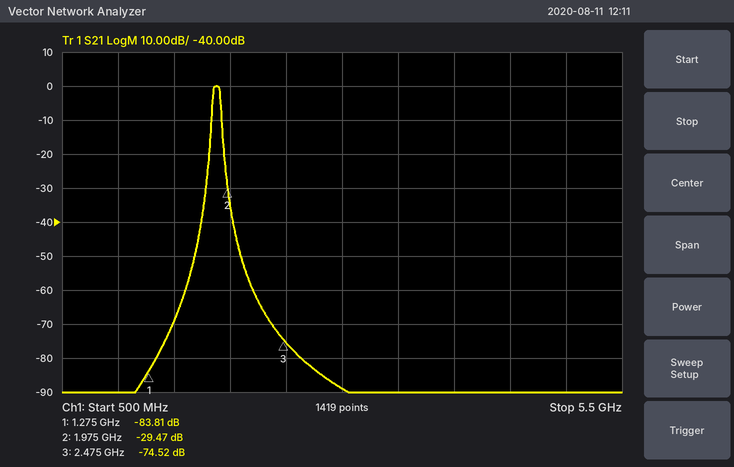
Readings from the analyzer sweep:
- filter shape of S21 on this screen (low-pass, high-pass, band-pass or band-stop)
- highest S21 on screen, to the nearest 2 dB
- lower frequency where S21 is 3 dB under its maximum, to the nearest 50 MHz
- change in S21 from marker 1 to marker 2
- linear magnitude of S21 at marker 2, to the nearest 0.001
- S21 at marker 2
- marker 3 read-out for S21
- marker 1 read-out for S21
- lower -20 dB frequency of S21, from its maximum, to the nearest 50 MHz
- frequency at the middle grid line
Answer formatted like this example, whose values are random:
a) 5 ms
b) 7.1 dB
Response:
a) band-pass
b) 0 dB
c) 1.85 GHz
d) 54.34 dB
e) 0.034
f) -29.47 dB
g) -74.52 dB
h) -83.81 dB
i) 1.80 GHz
j) 3 GHz
